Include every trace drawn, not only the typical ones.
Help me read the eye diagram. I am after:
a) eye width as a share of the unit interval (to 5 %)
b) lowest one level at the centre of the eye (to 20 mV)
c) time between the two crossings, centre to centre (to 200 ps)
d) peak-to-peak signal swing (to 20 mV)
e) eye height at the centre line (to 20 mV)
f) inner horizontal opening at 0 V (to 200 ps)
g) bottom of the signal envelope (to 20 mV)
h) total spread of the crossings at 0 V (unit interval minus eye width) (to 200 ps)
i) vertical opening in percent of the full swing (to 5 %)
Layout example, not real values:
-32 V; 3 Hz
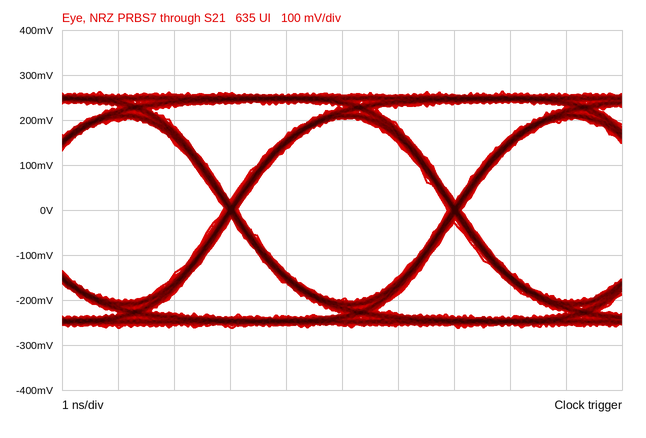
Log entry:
95 %; 200 mV; 4.0 ns; 520 mV; 400 mV; 3.8 ns; -260 mV; 200 ps; 75 %
